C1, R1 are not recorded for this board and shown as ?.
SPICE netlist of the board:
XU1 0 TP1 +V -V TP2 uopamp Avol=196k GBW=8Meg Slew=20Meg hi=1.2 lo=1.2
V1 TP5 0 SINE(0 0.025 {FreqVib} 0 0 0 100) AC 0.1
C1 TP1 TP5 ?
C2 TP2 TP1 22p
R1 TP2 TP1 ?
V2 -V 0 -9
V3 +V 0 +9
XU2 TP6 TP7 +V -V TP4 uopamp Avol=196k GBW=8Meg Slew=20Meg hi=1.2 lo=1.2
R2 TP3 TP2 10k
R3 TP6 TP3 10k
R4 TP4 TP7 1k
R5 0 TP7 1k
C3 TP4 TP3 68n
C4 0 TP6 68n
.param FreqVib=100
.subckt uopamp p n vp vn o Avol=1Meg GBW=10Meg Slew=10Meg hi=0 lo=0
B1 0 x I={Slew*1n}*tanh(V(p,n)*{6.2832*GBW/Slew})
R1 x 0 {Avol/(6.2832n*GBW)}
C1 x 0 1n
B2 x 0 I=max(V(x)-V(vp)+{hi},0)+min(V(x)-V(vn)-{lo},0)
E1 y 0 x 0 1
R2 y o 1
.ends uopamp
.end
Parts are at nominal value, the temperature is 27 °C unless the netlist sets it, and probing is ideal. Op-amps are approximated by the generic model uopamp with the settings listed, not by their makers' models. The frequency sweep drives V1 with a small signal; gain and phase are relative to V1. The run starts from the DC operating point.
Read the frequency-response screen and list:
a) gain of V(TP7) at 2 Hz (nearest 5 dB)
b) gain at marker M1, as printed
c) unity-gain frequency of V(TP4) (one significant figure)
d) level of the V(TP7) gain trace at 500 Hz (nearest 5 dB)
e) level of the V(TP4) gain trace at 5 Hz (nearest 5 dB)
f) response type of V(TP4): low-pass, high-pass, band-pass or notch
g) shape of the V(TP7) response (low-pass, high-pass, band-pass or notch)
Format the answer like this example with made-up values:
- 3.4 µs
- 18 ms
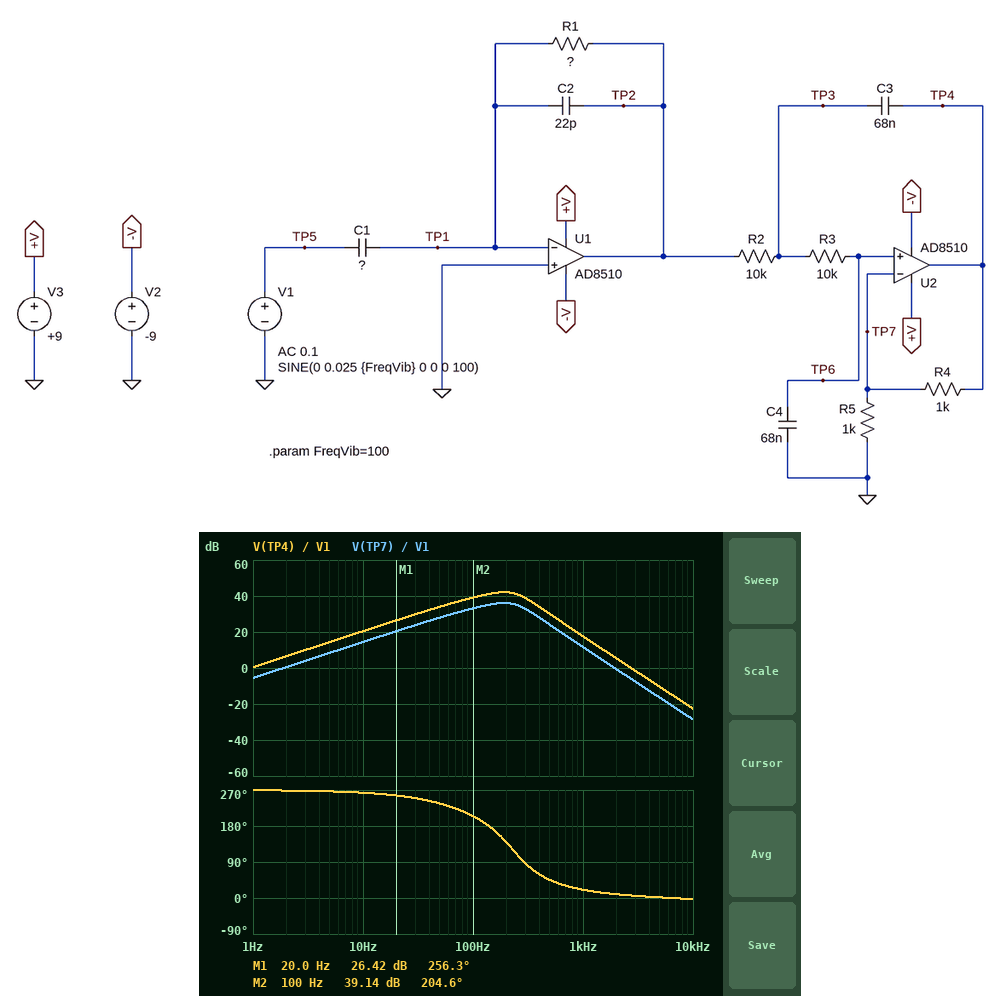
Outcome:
- 0 dB
- 26.42 dB
- 3 kHz
- 25 dB
- 15 dB
- band-pass
- band-pass
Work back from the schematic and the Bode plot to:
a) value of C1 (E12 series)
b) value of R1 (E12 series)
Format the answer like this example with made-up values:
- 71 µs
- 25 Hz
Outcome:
- 1.5 nF
- 56 MΩ
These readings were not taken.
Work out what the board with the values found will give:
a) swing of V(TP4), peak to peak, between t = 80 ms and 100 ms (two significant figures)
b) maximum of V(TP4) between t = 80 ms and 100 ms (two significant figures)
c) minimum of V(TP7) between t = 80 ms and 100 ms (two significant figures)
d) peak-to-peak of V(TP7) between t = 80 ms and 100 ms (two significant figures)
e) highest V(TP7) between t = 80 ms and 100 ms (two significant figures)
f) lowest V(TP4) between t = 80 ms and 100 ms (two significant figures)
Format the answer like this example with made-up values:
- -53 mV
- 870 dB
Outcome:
- 4.5 V
- 2.3 V
- -1.1 V
- 2.3 V
- 1.1 V
- -2.3 V
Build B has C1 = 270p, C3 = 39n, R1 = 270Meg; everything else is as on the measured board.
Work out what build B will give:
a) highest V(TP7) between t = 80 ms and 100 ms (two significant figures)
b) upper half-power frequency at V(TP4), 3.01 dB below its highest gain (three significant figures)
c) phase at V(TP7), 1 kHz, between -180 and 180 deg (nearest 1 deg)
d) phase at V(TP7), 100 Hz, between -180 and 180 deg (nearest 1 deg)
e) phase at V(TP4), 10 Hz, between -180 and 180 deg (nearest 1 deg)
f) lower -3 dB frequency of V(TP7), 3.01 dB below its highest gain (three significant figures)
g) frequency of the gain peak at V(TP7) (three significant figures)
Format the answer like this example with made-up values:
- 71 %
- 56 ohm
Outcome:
- 270 mV
- 250 Hz
- 34 deg
- 161 deg
- -114 deg
- 22.3 Hz
- 79.8 Hz
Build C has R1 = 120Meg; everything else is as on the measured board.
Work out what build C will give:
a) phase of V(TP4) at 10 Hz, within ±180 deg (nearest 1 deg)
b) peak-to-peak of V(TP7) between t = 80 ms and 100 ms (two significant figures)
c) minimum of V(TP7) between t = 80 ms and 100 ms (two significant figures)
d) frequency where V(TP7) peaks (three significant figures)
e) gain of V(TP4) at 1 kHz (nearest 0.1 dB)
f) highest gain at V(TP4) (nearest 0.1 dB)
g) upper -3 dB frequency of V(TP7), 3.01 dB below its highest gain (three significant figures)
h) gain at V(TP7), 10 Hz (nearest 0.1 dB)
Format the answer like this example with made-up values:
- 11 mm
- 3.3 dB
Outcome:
- -102 deg
- 3.2 V
- -1.6 V
- 177 Hz
- 17.7 dB
- 43.4 dB
- 280 Hz
- 21.0 dB
